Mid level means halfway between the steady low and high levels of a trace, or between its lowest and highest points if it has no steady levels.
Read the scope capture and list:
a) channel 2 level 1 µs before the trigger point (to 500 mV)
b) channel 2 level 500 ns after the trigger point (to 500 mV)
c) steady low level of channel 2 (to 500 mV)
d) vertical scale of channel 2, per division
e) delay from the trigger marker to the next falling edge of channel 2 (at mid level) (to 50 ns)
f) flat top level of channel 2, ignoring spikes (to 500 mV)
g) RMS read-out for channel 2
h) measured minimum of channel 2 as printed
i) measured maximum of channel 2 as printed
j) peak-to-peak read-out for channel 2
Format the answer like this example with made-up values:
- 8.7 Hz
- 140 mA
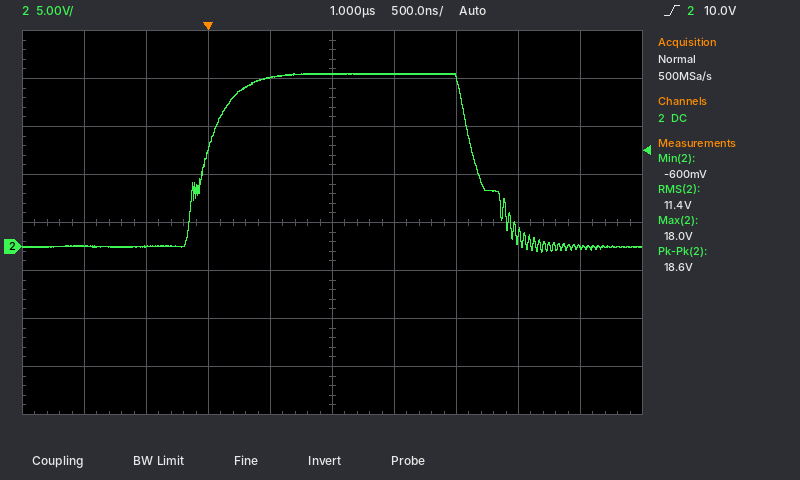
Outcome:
- 0.0 V
- 17.5 V
- 0.0 V
- 5 V
- 2.15 µs
- 18.0 V
- 11.4 V
- -600 mV
- 18.0 V
- 18.6 V
